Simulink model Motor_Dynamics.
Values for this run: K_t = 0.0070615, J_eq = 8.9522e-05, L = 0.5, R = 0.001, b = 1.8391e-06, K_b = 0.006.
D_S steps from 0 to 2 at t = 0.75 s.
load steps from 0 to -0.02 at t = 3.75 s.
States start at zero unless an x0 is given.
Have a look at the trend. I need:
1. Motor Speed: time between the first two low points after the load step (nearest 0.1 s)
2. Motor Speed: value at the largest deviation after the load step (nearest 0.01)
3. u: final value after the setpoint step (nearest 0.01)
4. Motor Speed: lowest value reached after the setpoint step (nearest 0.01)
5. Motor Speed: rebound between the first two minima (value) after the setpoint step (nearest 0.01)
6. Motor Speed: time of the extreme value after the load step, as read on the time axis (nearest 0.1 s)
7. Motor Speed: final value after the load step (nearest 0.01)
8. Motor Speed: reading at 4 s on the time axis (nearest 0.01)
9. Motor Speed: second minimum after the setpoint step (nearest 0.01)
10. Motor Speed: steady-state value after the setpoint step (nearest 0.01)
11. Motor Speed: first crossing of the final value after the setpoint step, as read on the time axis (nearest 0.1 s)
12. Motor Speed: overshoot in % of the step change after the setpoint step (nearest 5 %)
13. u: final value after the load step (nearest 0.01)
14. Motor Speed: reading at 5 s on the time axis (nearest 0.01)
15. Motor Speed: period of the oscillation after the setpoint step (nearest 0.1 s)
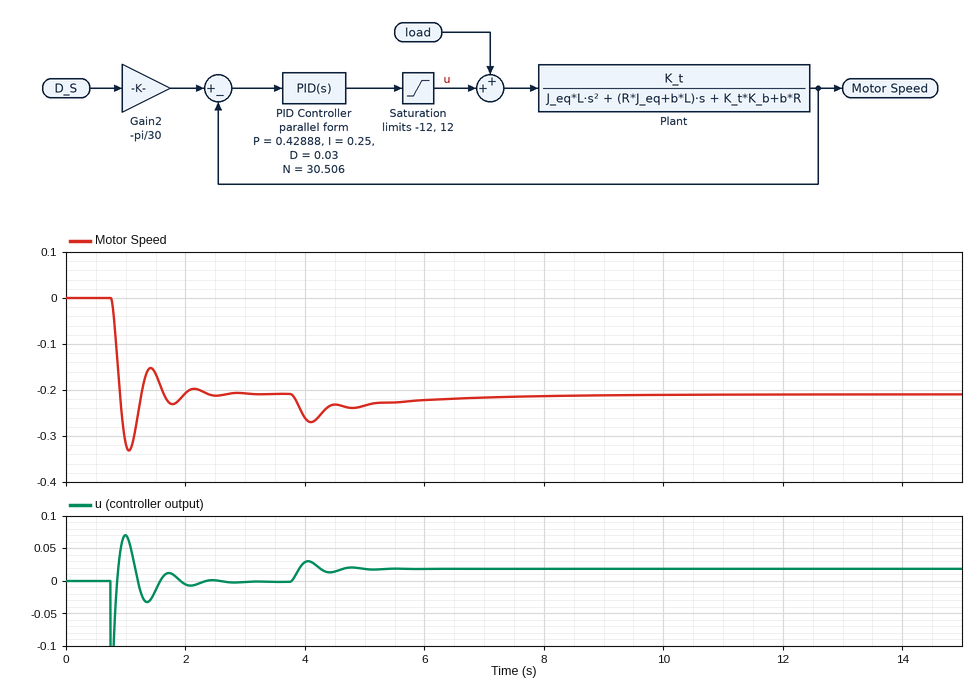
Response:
0.7 s
-0.27
0.00
-0.33
-0.15
4.1 s
-0.21
-0.26
-0.23
-0.21
0.9 s
60 %
0.02
-0.23
0.7 s
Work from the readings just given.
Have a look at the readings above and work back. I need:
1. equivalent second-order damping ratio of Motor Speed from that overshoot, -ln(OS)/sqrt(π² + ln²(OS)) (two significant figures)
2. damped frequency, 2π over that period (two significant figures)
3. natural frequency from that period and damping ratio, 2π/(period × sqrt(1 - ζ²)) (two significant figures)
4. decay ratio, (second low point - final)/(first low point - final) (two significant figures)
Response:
0.16
9.0 rad/s
9.1 rad/s
0.17
